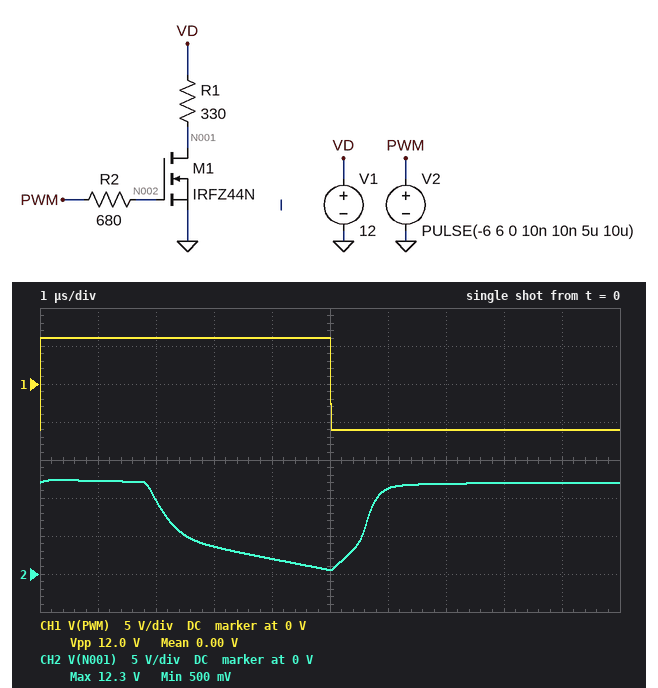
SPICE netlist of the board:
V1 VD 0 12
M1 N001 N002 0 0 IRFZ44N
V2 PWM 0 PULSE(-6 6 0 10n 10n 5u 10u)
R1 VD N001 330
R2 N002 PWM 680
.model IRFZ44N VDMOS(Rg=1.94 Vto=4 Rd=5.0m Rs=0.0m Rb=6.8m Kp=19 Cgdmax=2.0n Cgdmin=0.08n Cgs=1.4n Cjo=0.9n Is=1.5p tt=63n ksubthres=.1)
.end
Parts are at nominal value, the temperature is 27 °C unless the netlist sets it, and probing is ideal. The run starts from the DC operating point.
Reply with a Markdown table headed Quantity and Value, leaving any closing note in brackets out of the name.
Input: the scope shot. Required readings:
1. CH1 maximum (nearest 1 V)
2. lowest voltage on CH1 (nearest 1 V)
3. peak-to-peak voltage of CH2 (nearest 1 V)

| Quantity | Value |
|---|---|
| CH1 maximum | 6 V |
| lowest voltage on CH1 | -6 V |
| peak-to-peak voltage of CH2 | 12 V |
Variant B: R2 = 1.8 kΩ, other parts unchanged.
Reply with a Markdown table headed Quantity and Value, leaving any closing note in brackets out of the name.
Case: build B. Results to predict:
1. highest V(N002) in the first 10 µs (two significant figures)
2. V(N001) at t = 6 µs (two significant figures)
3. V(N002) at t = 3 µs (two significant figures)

| Quantity | Value |
|---|---|
| highest V(N002) in the first 10 µs | 3.9 V |
| V(N001) at t = 6 µs | 12 V |
| V(N002) at t = 3 µs | 1.9 V |
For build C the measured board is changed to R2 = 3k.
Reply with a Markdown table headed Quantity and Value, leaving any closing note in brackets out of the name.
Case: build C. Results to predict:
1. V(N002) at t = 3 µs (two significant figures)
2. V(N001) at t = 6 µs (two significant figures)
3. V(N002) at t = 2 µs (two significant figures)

| Quantity | Value |
|---|---|
| V(N002) at t = 3 µs | -250 mV |
| V(N001) at t = 6 µs | 12 V |
| V(N002) at t = 2 µs | -1.8 V |
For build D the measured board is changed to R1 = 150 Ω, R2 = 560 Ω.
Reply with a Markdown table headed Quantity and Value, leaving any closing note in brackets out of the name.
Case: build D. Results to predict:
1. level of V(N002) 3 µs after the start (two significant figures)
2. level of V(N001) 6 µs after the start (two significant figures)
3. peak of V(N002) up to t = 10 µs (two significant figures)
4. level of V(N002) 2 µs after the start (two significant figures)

| Quantity | Value |
|---|---|
| level of V(N002) 3 µs after the start | 4.0 V |
| level of V(N001) 6 µs after the start | 12 V |
| peak of V(N002) up to t = 10 µs | 4.5 V |
| level of V(N002) 2 µs after the start | 4.0 V |
